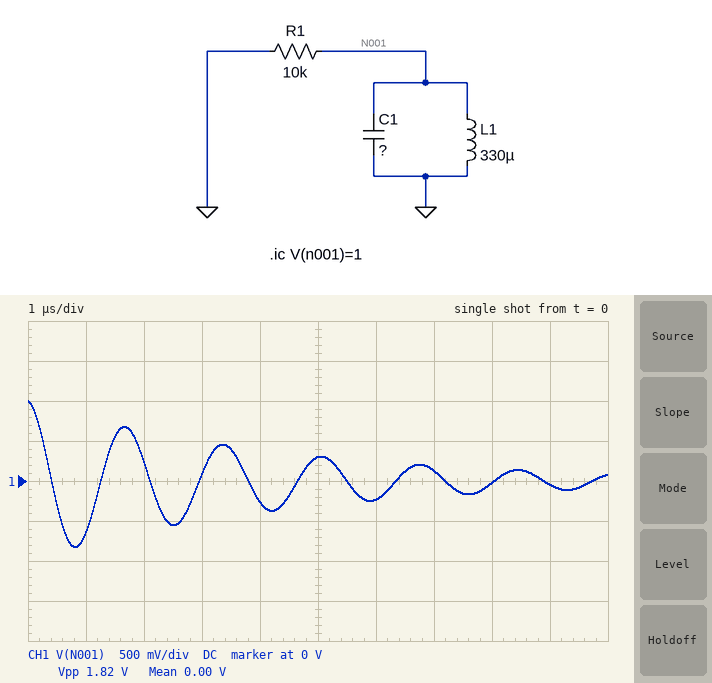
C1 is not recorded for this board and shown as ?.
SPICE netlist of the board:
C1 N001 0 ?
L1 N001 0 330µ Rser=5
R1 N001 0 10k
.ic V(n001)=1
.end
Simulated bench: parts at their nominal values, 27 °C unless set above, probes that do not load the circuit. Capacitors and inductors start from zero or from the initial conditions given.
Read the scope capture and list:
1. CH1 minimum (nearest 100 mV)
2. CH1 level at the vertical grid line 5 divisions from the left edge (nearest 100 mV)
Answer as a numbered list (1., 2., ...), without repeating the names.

1. -800 mV
2. 300 mV
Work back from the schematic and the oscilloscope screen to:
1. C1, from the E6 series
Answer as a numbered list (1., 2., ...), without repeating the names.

1. 220 pF
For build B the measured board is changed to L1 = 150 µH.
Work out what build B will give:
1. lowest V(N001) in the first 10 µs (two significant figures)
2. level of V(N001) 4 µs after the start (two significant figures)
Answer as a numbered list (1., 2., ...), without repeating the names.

1. -870 mV
2. -380 mV
